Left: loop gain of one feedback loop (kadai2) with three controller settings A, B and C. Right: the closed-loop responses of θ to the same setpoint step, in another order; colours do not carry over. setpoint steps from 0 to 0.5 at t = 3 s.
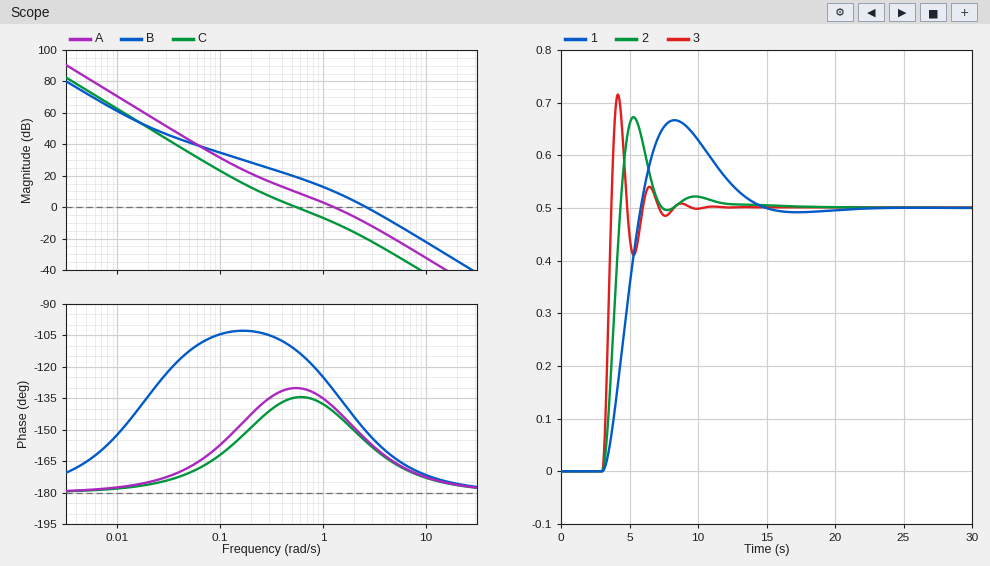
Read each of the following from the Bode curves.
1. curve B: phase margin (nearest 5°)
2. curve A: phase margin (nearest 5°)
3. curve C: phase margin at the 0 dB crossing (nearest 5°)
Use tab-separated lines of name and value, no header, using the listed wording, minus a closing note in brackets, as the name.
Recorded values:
curve B: phase margin	30°
curve A: phase margin	40°
curve C: phase margin at the 0 dB crossing	45°
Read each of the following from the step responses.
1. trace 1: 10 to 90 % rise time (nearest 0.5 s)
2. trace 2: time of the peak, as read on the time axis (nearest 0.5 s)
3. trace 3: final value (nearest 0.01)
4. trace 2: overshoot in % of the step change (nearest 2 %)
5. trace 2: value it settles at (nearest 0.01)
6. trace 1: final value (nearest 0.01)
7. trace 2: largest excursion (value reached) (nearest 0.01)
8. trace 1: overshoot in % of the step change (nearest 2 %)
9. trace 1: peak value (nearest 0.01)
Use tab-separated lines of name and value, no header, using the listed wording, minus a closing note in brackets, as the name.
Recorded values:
trace 1: 10 to 90 % rise time	2.0 s
trace 2: time of the peak, as read on the time axis	5.5 s
trace 3: final value	0.50
trace 2: overshoot in % of the step change	34 %
trace 2: value it settles at	0.50
trace 1: final value	0.50
trace 2: largest excursion (value reached)	0.67
trace 1: overshoot in % of the step change	34 %
trace 1: peak value	0.67
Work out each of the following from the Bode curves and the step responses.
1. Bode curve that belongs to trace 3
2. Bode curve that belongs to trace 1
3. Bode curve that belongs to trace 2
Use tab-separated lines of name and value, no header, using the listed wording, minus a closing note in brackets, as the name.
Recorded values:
Bode curve that belongs to trace 3	B
Bode curve that belongs to trace 1	C
Bode curve that belongs to trace 2	A
